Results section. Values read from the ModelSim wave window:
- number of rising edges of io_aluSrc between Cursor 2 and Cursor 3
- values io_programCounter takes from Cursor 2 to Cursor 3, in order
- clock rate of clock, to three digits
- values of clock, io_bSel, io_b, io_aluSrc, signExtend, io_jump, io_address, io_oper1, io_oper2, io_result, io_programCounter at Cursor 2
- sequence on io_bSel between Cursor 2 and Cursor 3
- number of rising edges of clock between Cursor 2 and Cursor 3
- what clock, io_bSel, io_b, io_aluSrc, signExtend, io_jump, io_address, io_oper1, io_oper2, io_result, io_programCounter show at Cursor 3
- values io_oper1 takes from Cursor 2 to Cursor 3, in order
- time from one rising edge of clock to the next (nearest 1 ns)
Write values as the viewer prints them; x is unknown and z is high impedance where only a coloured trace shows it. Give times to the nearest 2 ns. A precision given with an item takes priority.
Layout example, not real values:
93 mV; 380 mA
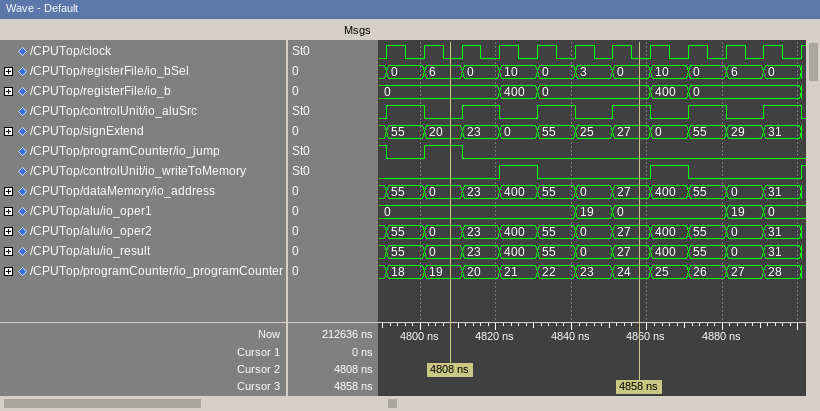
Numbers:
3; 19, 20, 21, 22, 23, 24; 100 MHz; clock=0, io_bSel=6, io_b=0, io_aluSrc=0, signExtend=20, io_jump=1, io_address=0, io_oper1=0, io_oper2=0, io_result=0, io_programCounter=19; 6, 0, 10, 0, 3, 0; 5; clock=0, io_bSel=0, io_b=0, io_aluSrc=1, signExtend=27, io_jump=0, io_address=27, io_oper1=0, io_oper2=27, io_result=27, io_programCounter=24; 0, 19, 0; 10 ns
